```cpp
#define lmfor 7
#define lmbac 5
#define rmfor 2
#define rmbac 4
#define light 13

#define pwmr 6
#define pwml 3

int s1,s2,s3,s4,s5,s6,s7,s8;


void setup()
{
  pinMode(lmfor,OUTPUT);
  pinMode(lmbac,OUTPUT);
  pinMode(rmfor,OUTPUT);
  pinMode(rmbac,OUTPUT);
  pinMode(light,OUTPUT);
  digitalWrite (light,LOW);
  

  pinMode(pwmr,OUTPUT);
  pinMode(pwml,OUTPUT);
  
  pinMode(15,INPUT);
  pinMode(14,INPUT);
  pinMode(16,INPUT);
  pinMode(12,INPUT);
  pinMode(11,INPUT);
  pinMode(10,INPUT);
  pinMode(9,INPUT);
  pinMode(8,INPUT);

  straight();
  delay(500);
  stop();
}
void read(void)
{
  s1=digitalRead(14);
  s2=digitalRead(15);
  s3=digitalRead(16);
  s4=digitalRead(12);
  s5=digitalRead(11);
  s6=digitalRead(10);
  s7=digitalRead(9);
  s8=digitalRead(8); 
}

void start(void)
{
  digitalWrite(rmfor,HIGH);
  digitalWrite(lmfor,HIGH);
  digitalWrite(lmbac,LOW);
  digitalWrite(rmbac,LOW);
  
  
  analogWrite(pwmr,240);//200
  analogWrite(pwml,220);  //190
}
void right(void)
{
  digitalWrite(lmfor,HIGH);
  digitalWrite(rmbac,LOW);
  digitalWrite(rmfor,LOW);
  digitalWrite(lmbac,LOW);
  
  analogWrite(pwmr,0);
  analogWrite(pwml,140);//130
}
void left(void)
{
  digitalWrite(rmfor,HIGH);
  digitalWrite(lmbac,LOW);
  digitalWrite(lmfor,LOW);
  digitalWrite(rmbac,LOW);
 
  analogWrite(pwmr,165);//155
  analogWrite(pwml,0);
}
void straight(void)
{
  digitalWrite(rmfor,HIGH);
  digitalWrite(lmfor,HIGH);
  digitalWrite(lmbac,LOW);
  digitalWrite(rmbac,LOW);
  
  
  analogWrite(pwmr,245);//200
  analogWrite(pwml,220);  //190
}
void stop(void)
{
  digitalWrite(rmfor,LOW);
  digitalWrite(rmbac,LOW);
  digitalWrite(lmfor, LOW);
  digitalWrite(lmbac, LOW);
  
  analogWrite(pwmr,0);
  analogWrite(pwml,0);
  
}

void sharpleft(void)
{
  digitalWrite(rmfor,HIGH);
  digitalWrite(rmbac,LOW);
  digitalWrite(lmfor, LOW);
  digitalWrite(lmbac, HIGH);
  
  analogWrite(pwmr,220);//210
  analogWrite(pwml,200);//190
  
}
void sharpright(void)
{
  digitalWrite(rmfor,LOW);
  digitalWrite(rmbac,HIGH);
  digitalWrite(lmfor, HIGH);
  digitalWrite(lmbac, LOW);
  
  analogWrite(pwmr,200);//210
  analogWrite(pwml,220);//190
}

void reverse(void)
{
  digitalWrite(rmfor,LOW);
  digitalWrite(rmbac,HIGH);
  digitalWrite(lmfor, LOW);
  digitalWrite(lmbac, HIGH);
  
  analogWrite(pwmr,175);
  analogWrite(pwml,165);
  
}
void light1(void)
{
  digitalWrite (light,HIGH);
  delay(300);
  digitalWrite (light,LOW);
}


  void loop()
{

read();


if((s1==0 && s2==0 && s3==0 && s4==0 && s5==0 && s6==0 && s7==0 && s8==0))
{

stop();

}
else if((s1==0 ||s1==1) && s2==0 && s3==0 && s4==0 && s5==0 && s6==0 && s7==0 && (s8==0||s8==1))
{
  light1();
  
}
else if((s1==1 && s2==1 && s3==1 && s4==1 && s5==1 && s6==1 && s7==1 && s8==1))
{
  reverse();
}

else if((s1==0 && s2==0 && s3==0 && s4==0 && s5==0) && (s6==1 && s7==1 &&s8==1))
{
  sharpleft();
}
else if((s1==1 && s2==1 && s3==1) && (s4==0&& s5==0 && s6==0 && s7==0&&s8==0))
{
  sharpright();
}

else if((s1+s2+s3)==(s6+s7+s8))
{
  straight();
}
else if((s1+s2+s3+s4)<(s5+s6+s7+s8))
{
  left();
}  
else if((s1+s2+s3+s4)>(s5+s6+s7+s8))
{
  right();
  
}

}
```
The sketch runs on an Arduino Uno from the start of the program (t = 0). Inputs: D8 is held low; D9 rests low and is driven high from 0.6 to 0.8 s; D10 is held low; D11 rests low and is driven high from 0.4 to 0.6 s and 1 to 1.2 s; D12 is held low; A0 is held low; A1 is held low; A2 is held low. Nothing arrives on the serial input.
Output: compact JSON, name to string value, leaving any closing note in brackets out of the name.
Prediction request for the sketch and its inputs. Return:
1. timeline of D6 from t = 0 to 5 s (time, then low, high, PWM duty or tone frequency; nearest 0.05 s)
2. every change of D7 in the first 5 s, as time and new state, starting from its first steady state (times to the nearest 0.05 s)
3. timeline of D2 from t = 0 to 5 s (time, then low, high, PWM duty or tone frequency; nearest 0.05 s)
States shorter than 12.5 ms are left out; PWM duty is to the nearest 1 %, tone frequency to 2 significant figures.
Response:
{"timeline of D6 from t = 0 to 5 s": "0 s PWM 96 %; 0.6 s PWM 65 %; 0.8 s low; 1 s PWM 96 %; 1.2 s low", "every change of D7 in the first 5 s, as time and new state, starting from its first steady state": "0 s high; 0.6 s low; 1 s high; 1.2 s low", "timeline of D2 from t = 0 to 5 s": "0 s high; 0.8 s low; 1 s high; 1.2 s low"}
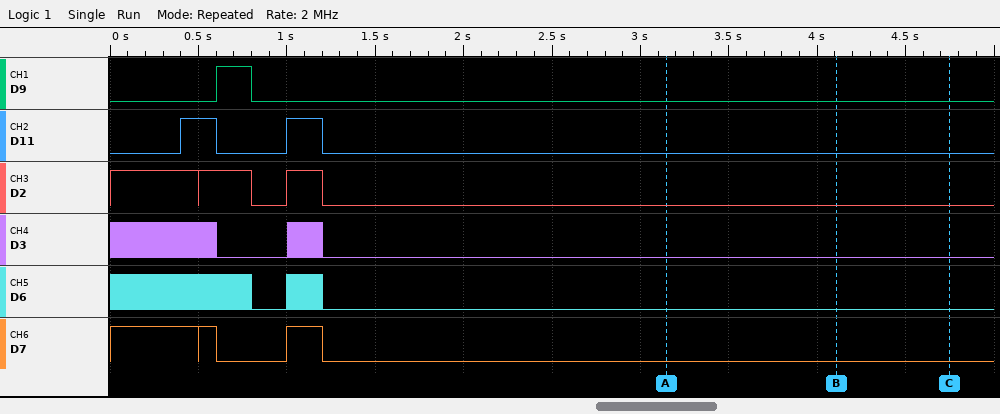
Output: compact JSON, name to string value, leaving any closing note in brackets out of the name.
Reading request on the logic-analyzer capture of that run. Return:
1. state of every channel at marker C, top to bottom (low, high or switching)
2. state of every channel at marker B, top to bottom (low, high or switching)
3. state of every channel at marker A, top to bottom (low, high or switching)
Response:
{"state of every channel at marker C, top to bottom": "D9 low, D11 low, D2 low, D3 low, D6 low, D7 low", "state of every channel at marker B, top to bottom": "D9 low, D11 low, D2 low, D3 low, D6 low, D7 low", "state of every channel at marker A, top to bottom": "D9 low, D11 low, D2 low, D3 low, D6 low, D7 low"}
